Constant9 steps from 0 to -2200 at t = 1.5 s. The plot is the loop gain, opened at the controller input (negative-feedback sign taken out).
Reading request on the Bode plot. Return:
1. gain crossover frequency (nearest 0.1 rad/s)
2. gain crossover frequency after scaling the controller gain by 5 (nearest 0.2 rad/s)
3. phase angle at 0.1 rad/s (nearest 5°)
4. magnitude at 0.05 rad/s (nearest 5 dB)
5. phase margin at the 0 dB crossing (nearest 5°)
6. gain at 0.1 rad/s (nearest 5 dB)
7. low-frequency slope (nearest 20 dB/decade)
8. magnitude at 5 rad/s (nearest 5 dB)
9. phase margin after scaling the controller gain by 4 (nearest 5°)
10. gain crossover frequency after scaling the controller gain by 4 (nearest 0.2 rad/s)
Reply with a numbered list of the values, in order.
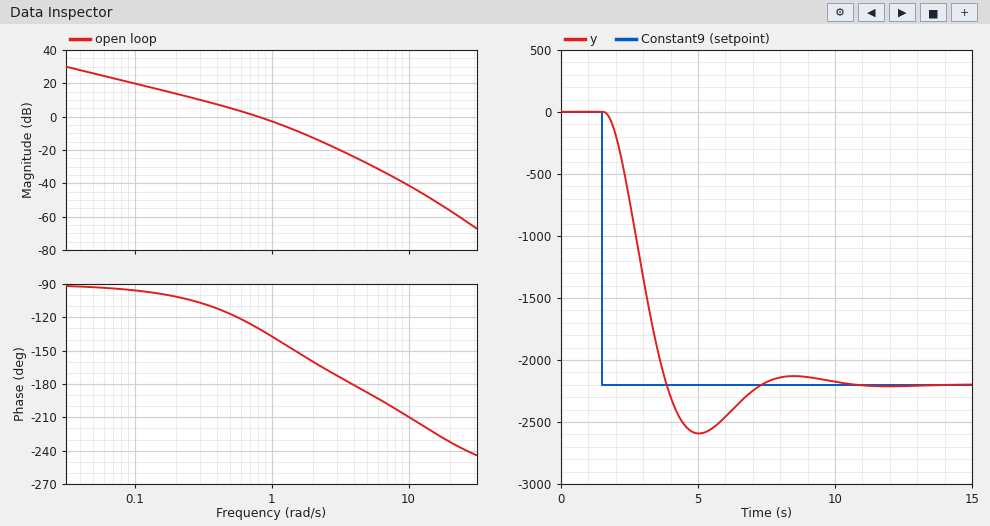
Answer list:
1. 0.8 rad/s
2. 2.2 rad/s
3. -95°
4. 25 dB
5. 50°
6. 20 dB
7. -20 dB/decade
8. -30 dB
9. 20°
10. 2.0 rad/s
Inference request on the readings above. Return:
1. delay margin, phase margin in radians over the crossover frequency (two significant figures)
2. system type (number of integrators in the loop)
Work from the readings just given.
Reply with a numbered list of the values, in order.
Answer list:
1. 1.1 s
2. 1
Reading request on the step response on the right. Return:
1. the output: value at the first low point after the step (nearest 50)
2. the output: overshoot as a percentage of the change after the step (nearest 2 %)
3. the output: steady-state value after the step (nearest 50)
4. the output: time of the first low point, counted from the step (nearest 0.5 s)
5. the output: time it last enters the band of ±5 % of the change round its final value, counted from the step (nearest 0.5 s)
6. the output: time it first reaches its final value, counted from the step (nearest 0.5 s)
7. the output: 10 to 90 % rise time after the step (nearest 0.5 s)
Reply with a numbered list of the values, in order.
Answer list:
1. -2600
2. 18 %
3. -2200
4. 3.5 s
5. 5.0 s
6. 2.5 s
7. 1.5 s
